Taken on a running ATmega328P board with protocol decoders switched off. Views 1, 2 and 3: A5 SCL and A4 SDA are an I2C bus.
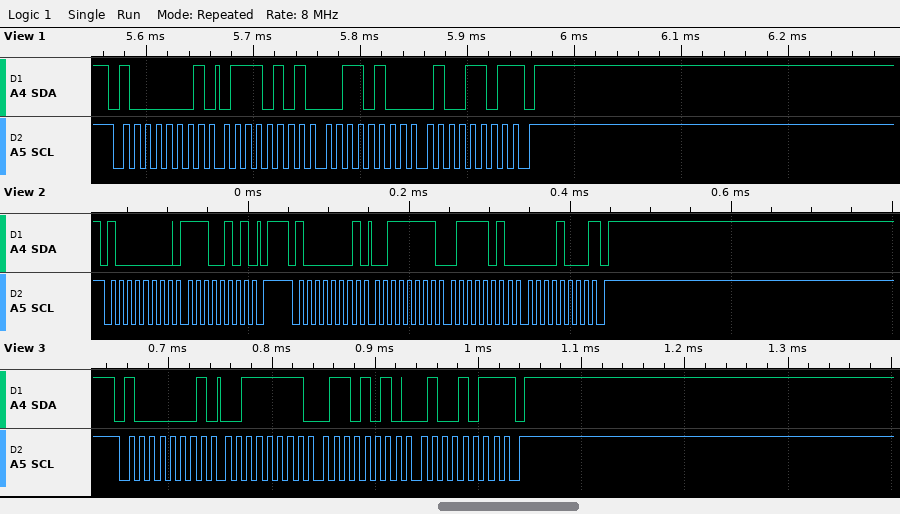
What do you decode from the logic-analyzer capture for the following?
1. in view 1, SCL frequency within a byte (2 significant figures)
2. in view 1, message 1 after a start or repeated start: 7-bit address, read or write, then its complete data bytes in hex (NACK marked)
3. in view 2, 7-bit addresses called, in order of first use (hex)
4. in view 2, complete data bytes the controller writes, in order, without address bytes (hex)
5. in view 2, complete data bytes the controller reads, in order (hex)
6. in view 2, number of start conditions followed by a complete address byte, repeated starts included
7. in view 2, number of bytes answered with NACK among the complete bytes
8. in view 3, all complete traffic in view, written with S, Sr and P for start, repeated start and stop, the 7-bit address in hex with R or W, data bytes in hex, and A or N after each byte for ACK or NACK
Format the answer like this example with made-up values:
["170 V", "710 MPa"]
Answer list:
["100 kHz", "0x40 read: 75 34 4D NACK", "0x40", "E5", "3F 7A 08", "2", "1", "S 40R A 3F A 6A A 4B N P"]
